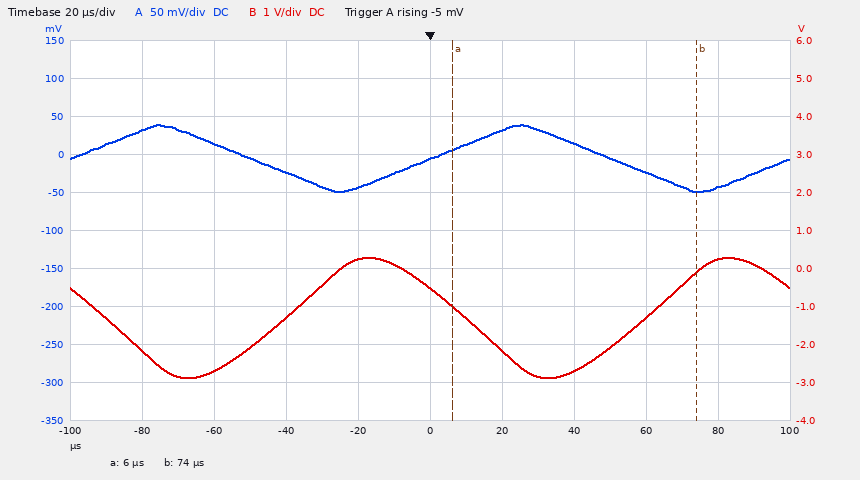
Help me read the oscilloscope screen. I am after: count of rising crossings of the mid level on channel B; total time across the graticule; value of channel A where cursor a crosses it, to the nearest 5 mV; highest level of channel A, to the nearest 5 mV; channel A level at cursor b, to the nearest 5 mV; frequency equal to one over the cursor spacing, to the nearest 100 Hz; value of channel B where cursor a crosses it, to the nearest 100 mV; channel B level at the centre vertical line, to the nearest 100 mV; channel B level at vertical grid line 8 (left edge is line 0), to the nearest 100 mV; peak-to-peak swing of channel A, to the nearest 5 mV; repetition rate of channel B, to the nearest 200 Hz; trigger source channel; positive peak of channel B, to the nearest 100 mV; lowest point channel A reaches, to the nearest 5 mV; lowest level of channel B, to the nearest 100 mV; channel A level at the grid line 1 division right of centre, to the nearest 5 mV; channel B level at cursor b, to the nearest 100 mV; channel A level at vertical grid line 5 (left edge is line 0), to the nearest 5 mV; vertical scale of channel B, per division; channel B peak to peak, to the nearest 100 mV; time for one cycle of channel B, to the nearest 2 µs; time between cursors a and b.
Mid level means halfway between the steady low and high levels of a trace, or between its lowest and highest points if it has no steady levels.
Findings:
2
200 µs
5 mV
40 mV
-50 mV
14.7 kHz
-1.0 V
-500 mV
-1.3 V
90 mV
10.0 kHz
channel A
300 mV
-50 mV
-2.9 V
30 mV
-100 mV
-5 mV
1 V
3.2 V
100 µs
68 µs
